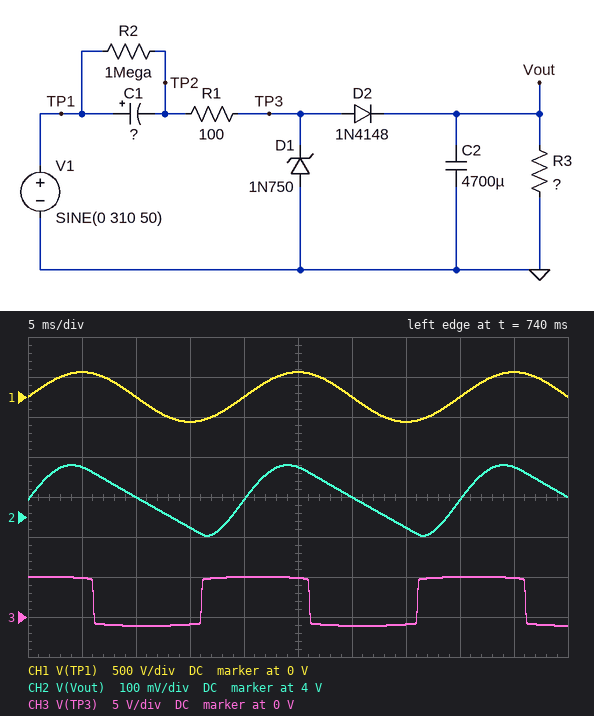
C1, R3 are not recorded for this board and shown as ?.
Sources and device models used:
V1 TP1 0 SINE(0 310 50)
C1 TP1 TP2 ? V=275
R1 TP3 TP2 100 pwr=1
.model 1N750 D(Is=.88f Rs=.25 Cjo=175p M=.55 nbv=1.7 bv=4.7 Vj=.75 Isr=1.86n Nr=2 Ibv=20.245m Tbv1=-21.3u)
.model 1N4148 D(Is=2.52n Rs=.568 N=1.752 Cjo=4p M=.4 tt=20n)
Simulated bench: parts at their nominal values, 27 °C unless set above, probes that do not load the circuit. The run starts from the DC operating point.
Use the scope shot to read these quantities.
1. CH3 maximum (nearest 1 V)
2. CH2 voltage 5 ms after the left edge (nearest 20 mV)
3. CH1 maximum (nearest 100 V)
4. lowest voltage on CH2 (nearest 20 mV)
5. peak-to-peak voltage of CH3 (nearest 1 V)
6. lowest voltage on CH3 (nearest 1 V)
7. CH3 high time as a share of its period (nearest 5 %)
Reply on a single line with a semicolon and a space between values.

5 V; 4.12 V; 300 V; 3.96 V; 6 V; -1 V; 50 %
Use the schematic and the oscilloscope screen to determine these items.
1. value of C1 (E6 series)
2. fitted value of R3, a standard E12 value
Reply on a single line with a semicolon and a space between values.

10 µF; 56 Ω
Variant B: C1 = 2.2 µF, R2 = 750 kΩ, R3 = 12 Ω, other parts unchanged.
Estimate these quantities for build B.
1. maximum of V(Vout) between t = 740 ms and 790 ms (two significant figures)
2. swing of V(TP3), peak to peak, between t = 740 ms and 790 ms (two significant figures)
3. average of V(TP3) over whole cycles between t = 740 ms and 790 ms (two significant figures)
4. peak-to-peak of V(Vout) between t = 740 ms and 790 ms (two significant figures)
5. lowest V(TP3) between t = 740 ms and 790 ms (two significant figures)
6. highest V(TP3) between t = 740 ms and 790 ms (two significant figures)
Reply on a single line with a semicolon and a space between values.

890 mV; 2.7 V; 410 mV; 160 mV; -910 mV; 1.8 V
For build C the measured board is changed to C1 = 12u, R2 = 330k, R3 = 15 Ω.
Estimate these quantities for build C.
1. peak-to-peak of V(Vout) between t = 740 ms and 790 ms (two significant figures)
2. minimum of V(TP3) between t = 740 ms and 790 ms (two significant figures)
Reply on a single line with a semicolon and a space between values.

550 mV; -1.2 V
